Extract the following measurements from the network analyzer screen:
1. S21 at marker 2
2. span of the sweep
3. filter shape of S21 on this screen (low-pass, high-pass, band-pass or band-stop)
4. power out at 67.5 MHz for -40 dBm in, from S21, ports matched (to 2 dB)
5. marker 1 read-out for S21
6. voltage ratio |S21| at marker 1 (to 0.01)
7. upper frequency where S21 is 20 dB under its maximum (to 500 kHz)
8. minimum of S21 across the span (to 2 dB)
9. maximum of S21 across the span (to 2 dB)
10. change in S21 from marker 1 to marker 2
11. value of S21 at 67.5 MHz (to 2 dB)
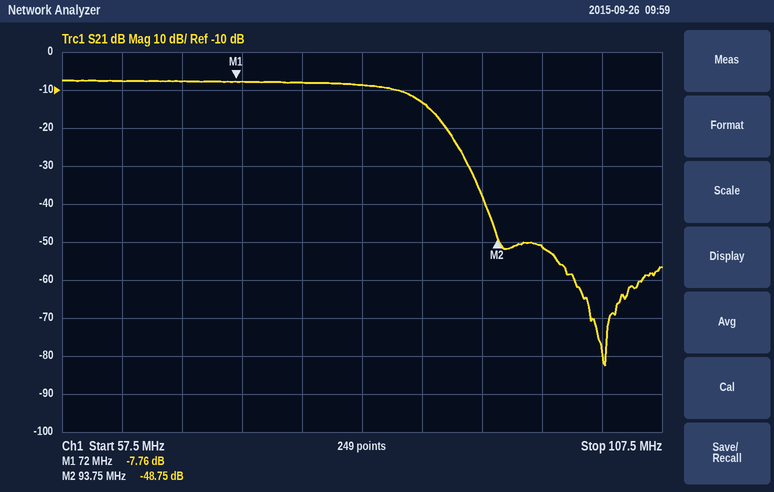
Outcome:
-48.75 dB
50 MHz
low-pass
-48 dBm
-7.76 dB
0.41
91.0 MHz
-82 dB
-8 dB
-40.99 dB
-8 dB
